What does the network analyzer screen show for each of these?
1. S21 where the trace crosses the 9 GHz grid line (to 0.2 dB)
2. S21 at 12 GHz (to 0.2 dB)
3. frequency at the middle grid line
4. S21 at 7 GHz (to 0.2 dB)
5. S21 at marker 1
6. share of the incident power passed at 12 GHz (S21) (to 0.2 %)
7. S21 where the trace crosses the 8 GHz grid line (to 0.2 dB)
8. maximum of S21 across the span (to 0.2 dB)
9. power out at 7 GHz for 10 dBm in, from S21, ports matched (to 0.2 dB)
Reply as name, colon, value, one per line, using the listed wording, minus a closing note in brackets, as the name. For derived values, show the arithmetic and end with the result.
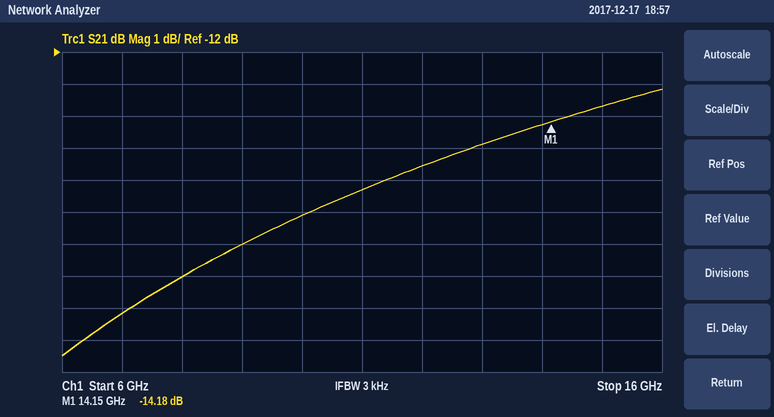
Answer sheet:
S21 where the trace crosses the 9 GHz grid line: -18.0 dB
S21 at 12 GHz: -15.6 dB
frequency at the middle grid line: 11 GHz
S21 at 7 GHz: -20.2 dB
S21 at marker 1: -14.18 dB
share of the incident power passed at 12 GHz (S21): 10^(-15.6/10) ≈ 2.8 %
S21 where the trace crosses the 8 GHz grid line: -19.0 dB
maximum of S21 across the span: -13.2 dB
power out at 7 GHz for 10 dBm in, from S21, ports matched: 10 dBm + (-20.2 dB) = -10.2 dBm
